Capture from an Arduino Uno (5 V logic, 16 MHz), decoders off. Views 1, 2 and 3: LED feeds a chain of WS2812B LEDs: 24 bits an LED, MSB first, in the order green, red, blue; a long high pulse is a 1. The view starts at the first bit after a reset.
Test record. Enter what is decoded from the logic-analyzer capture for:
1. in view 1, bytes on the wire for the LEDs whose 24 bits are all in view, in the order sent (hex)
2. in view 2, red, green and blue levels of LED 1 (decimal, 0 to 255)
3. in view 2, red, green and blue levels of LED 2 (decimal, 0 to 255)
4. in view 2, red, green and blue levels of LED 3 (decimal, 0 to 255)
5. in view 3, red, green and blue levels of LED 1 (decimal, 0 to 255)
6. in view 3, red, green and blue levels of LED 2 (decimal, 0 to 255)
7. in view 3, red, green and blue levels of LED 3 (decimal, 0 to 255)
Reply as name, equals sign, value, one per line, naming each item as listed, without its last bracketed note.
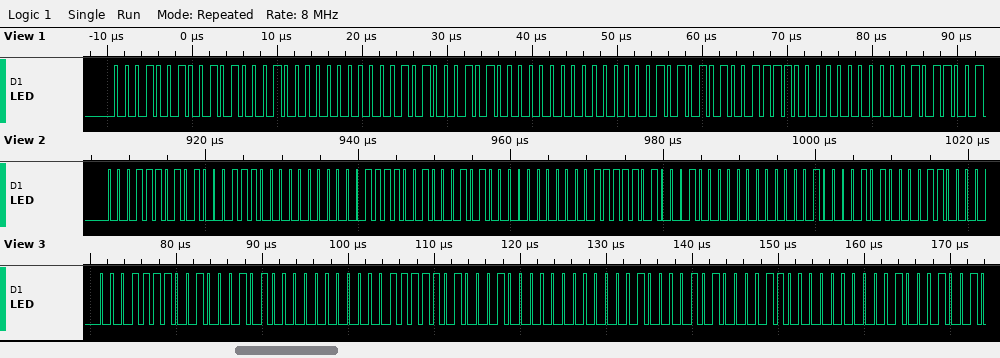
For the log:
in view 1, bytes on the wire for the LEDs whose 24 bits are all in view, in the order sent = 12 51 00 14 50 00 15 4F 00
in view 2, red, green and blue levels of LED 1 = 71, 29, 0
in view 2, red, green and blue levels of LED 2 = 69, 30, 0
in view 2, red, green and blue levels of LED 3 = 68, 31, 0
in view 3, red, green and blue levels of LED 1 = 69, 30, 0
in view 3, red, green and blue levels of LED 2 = 68, 31, 0
in view 3, red, green and blue levels of LED 3 = 67, 33, 0
